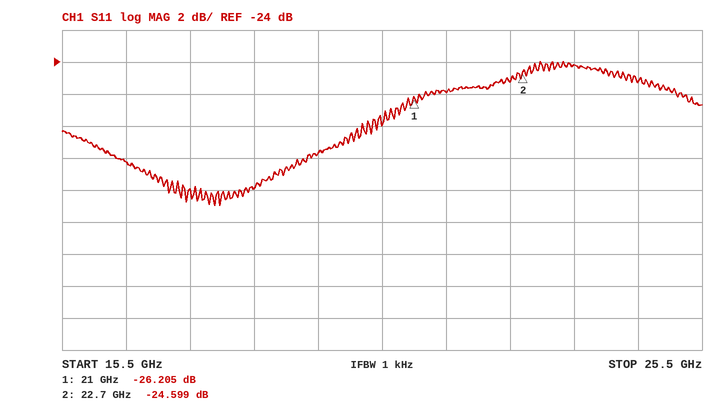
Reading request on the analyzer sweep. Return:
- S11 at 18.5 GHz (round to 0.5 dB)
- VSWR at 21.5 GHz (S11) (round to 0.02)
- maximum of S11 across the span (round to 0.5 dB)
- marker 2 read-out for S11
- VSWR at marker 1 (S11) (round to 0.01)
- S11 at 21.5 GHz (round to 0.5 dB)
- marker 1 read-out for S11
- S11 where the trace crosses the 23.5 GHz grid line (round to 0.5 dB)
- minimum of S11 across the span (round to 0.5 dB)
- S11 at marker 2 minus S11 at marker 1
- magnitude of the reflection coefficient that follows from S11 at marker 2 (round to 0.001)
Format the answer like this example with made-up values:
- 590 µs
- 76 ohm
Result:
- -32.0 dB
- 1.10
- -24.0 dB
- -24.599 dB
- 1.10
- -26.0 dB
- -26.205 dB
- -24.0 dB
- -33.0 dB
- 1.606 dB
- 0.059
